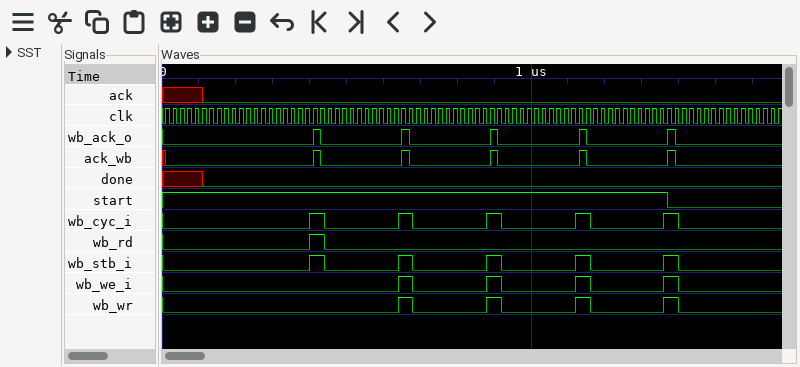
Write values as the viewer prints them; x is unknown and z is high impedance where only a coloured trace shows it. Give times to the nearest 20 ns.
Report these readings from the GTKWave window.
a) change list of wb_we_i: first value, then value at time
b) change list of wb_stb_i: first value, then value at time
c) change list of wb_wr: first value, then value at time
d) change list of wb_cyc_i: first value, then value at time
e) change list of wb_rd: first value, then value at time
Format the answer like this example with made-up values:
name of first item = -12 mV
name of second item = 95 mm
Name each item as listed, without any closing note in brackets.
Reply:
change list of wb_we_i: first value, then value at time = 0, 1 at 640 ns, 0 at 680 ns, 1 at 880 ns, 0 at 920 ns, 1 at 1120 ns, 0 at 1160 ns, 1 at 1360 ns, 0 at 1400 ns
change list of wb_stb_i: first value, then value at time = 0, 1 at 400 ns, 0 at 440 ns, 1 at 640 ns, 0 at 680 ns, 1 at 880 ns, 0 at 920 ns, 1 at 1120 ns, 0 at 1160 ns, 1 at 1360 ns, 0 at 1400 ns
change list of wb_wr: first value, then value at time = 0, 1 at 640 ns, 0 at 680 ns, 1 at 880 ns, 0 at 920 ns, 1 at 1120 ns, 0 at 1160 ns, 1 at 1360 ns, 0 at 1400 ns
change list of wb_cyc_i: first value, then value at time = 0, 1 at 400 ns, 0 at 440 ns, 1 at 640 ns, 0 at 680 ns, 1 at 880 ns, 0 at 920 ns, 1 at 1120 ns, 0 at 1160 ns, 1 at 1360 ns, 0 at 1400 ns
change list of wb_rd: first value, then value at time = 0, 1 at 400 ns, 0 at 440 ns
